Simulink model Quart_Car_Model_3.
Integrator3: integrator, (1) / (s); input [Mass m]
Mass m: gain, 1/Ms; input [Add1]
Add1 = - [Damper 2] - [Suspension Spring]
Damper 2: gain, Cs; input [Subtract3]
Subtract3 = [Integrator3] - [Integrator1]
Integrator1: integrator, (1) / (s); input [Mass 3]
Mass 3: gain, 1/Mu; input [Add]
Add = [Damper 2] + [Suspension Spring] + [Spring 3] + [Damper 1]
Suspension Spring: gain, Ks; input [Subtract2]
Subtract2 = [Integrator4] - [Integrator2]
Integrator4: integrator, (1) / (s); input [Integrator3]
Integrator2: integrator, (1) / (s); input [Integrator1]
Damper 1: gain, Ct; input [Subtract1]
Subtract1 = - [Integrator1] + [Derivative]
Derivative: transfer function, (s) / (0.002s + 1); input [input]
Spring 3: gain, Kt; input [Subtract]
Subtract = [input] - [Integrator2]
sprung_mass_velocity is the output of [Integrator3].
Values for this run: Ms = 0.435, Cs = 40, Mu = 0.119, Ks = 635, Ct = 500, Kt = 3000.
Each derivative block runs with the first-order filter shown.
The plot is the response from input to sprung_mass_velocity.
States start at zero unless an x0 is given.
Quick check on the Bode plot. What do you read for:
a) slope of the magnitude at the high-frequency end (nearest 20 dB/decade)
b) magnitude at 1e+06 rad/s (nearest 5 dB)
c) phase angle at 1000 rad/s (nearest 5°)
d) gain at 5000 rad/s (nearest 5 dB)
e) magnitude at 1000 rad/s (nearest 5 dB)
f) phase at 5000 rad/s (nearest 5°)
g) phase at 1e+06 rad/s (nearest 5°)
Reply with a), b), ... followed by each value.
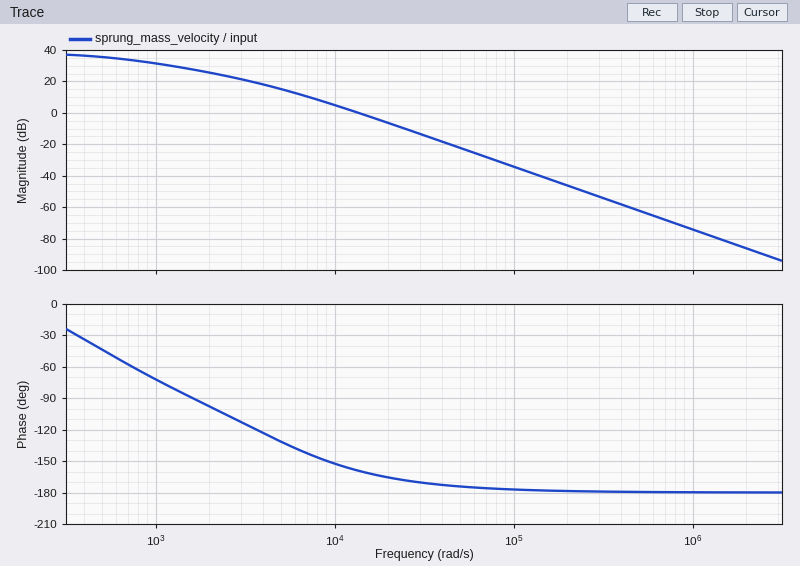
a) -40 dB/decade
b) -75 dB
c) -70°
d) 15 dB
e) 30 dB
f) -130°
g) -180°
